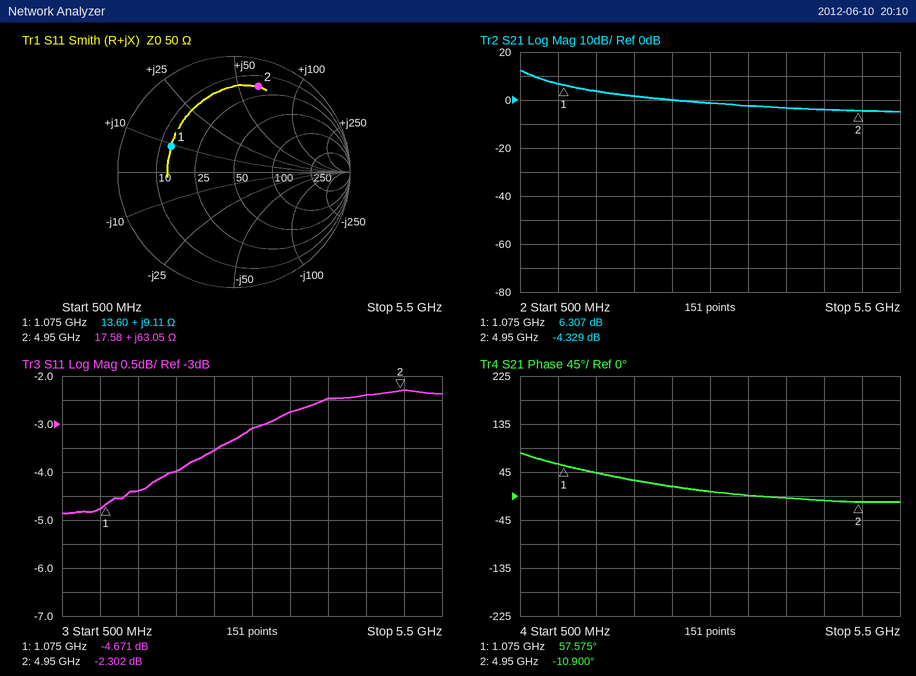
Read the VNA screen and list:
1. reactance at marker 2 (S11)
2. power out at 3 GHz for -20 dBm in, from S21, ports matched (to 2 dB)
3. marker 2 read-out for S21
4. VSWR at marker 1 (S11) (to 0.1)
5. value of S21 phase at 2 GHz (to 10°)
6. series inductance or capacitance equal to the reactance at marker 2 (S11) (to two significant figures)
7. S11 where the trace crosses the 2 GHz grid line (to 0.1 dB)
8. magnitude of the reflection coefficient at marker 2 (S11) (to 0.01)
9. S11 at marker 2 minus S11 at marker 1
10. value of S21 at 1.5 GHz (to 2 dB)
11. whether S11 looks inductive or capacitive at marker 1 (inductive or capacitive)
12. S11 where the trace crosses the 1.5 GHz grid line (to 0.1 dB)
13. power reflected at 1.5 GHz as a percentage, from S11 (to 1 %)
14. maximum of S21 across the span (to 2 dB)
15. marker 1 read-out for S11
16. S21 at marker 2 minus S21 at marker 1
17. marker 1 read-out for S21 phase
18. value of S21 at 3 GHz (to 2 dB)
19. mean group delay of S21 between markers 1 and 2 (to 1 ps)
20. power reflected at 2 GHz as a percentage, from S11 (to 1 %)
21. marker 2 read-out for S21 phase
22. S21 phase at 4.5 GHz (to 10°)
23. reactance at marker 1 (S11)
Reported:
+63.05 Ω
-22 dBm
-4.329 dB
3.8
30°
2.0 nH
-4.0 dB
0.77
2.369 dB
4 dB
inductive
-4.4 dB
36 %
12 dB
-4.671 dB
-10.636 dB
57.575°
-2 dB
49 ps
40 %
-10.900°
-10°
+9.11 Ω
